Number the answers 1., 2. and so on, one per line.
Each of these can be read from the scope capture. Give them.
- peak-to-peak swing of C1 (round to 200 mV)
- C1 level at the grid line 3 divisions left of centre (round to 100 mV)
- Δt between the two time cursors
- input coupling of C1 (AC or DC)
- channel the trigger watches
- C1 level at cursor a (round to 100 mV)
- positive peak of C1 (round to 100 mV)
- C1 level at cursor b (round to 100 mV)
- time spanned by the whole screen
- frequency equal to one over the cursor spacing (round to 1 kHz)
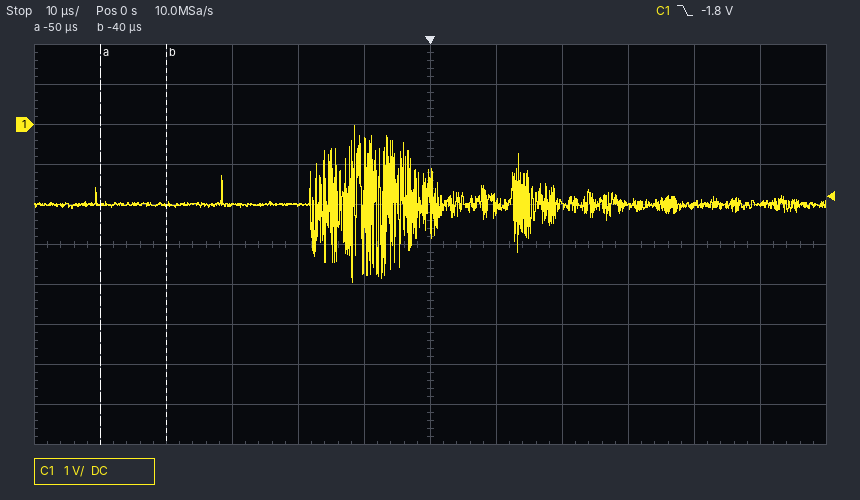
1. 4.0 V
2. -2.0 V
3. 10 µs
4. DC
5. C1
6. -2.0 V
7. 0.0 V
8. -2.0 V
9. 120 µs
10. 100 kHz
